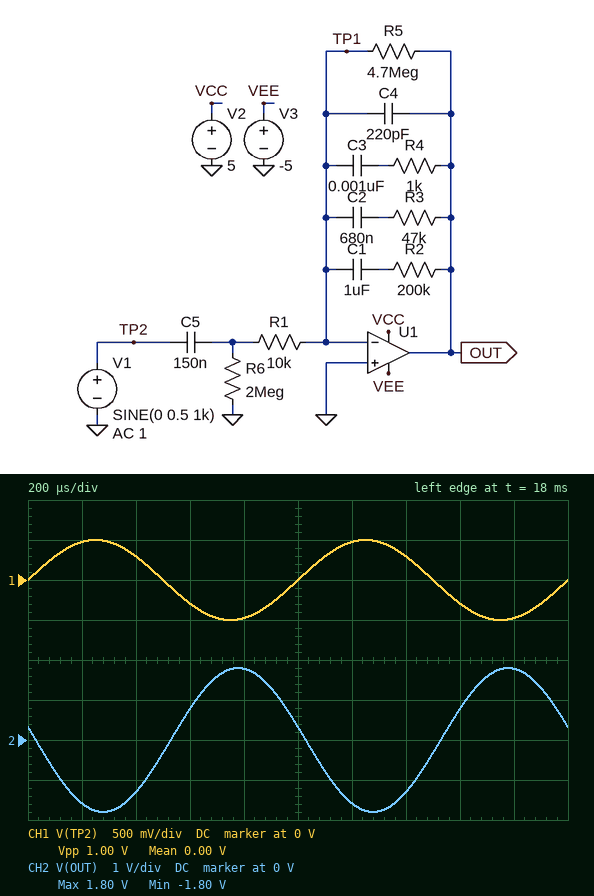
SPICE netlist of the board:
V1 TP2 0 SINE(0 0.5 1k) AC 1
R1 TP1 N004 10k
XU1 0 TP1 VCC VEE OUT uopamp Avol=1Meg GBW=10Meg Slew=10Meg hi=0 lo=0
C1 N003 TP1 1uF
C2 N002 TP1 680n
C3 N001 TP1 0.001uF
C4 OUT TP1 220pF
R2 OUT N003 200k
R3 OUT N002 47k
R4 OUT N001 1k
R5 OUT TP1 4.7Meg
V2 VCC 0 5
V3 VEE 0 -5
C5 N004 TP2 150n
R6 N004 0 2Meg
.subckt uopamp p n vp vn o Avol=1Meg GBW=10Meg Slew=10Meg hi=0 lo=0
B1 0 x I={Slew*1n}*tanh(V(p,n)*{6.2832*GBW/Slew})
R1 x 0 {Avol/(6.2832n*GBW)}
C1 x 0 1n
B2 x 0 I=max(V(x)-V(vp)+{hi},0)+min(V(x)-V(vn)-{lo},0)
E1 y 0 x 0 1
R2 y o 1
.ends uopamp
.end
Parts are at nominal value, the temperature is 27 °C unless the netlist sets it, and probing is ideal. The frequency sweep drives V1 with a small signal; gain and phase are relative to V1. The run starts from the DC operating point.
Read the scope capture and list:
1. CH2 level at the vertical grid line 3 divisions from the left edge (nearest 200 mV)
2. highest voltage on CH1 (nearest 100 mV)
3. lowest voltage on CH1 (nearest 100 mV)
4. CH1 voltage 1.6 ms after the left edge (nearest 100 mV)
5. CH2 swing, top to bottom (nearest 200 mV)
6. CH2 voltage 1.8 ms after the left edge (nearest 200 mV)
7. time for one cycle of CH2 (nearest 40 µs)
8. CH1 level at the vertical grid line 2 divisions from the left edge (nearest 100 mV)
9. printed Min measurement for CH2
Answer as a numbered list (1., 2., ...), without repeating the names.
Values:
1. 800 mV
2. 500 mV
3. -500 mV
4. -300 mV
5. 3.6 V
6. 1.8 V
7. 1.00 ms
8. 300 mV
9. -1.80 V
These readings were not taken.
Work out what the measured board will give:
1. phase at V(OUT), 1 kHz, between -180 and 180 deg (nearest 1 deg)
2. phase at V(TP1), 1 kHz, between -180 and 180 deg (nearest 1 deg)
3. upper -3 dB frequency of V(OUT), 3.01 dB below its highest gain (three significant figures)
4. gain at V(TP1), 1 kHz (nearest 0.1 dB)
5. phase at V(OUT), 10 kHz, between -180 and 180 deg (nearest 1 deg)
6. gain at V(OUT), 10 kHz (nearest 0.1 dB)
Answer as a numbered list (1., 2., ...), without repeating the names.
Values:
1. 170 deg
2. 79 deg
3. 3.60 kHz
4. -68.9 dB
5. 112 deg
6. 1.7 dB
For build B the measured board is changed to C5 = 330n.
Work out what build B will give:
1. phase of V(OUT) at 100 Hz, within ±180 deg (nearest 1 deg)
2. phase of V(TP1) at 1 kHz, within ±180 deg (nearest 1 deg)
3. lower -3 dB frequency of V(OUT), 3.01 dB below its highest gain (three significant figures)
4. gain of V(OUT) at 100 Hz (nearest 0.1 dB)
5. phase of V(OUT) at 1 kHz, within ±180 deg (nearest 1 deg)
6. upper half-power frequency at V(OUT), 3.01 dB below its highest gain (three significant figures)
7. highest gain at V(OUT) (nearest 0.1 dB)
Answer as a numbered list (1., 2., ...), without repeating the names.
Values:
1. -158 deg
2. 76 deg
3. 46.7 Hz
4. 10.6 dB
5. 166 deg
6. 3.49 kHz
7. 11.4 dB
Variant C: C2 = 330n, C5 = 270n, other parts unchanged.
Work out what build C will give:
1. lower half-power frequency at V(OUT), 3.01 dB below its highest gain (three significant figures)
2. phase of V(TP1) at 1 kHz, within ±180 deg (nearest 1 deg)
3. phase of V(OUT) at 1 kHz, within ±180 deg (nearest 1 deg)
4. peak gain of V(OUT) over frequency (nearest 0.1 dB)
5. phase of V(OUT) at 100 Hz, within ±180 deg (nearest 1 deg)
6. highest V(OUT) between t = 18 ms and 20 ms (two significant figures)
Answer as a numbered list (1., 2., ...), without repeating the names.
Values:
1. 55.6 Hz
2. 76 deg
3. 167 deg
4. 11.4 dB
5. -156 deg
6. 1.8 V
